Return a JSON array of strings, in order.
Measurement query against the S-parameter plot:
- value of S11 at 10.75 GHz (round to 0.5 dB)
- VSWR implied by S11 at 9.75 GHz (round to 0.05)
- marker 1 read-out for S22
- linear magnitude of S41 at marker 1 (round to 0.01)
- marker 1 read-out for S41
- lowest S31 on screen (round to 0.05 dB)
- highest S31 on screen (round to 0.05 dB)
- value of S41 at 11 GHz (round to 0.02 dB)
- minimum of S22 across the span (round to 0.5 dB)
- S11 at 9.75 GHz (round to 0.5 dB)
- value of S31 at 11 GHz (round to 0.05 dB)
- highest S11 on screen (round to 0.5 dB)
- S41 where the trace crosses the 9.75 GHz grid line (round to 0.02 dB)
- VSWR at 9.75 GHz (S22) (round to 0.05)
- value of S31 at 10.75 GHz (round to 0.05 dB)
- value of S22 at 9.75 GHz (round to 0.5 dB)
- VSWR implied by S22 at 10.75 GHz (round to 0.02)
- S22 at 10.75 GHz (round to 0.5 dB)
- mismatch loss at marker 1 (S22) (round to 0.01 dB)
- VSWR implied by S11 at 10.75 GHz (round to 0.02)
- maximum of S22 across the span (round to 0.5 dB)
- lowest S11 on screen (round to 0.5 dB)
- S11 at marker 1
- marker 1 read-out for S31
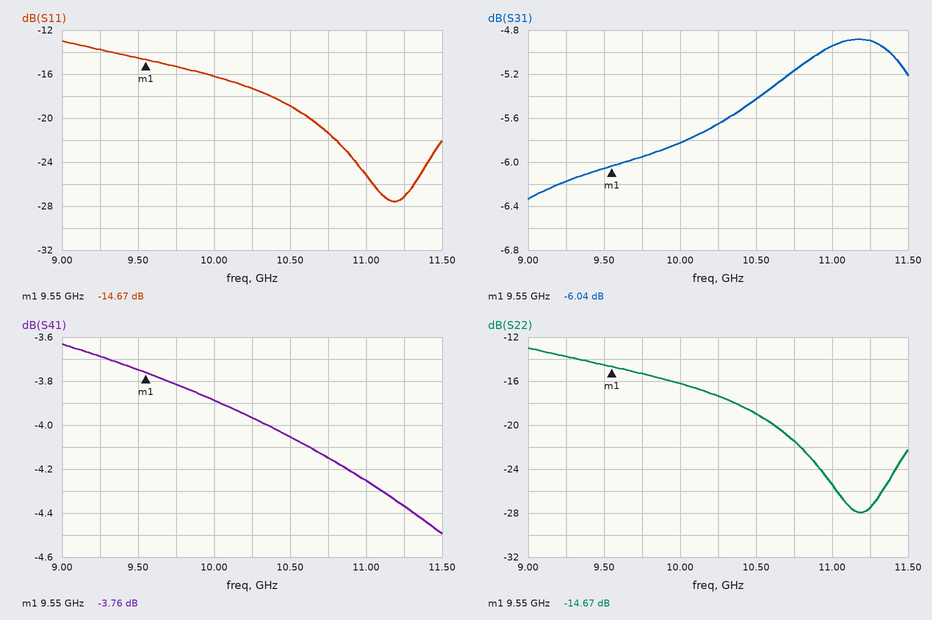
["-21.5 dB", "1.40", "-14.67 dB", "0.65", "-3.76 dB", "-6.35 dB", "-4.90 dB", "-4.26 dB", "-28.0 dB", "-15.5 dB", "-4.95 dB", "-13.0 dB", "-3.82 dB", "1.40", "-5.15 dB", "-15.5 dB", "1.18", "-21.5 dB", "0.15 dB", "1.18", "-13.0 dB", "-27.5 dB", "-14.67 dB", "-6.04 dB"]
